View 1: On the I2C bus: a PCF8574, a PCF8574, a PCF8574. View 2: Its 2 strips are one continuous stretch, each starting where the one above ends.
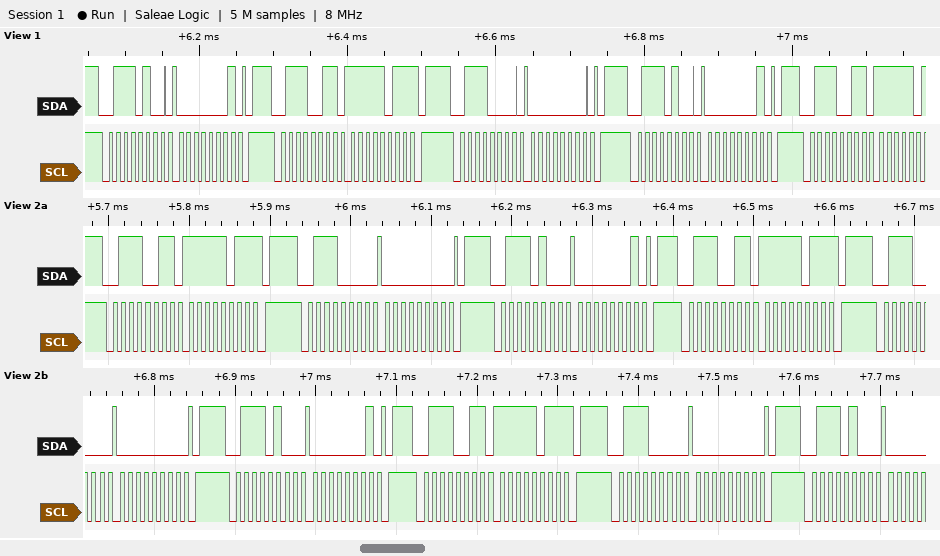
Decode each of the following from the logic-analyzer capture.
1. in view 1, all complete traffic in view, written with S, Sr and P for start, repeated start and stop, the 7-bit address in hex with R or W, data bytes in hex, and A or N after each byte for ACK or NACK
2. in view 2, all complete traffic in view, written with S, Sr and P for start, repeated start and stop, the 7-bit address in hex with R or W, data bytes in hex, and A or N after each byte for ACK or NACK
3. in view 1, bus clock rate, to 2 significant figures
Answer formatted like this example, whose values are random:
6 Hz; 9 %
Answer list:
S 3AW A 01 A P S 39R A FB N P S 38W A 00 A P S 3AW A 01 A P S 39R A; S 39R A FB N P S 38W A 00 A P S 3AW A 01 A P S 39R A FB N P S 38W A 00 A P S 3AW A 01 A P S 39R A FB N P S 38W A 00 A P S 3AW A; 100 kHz
